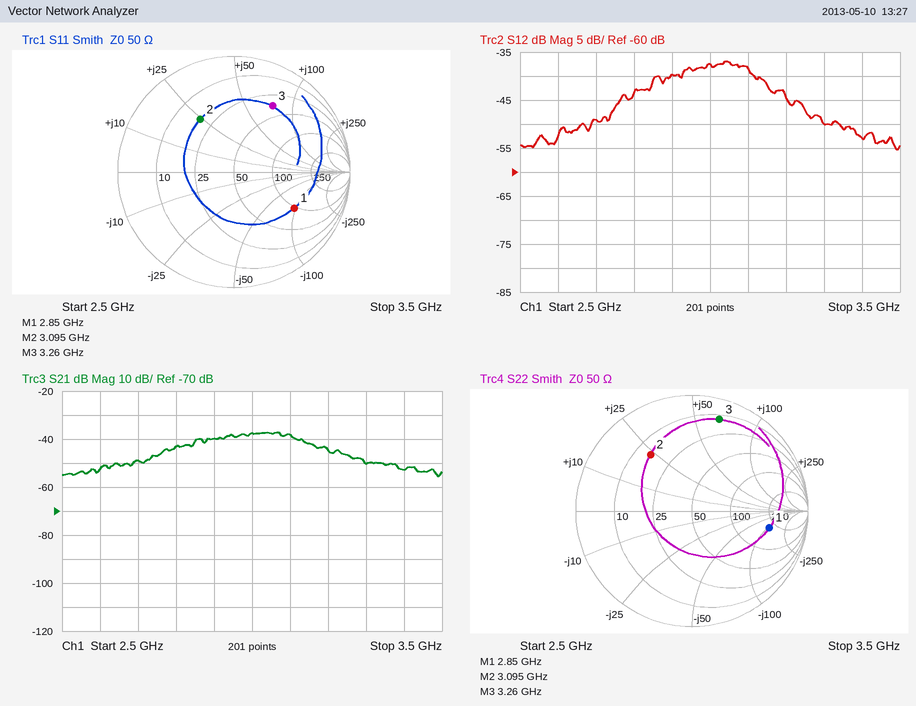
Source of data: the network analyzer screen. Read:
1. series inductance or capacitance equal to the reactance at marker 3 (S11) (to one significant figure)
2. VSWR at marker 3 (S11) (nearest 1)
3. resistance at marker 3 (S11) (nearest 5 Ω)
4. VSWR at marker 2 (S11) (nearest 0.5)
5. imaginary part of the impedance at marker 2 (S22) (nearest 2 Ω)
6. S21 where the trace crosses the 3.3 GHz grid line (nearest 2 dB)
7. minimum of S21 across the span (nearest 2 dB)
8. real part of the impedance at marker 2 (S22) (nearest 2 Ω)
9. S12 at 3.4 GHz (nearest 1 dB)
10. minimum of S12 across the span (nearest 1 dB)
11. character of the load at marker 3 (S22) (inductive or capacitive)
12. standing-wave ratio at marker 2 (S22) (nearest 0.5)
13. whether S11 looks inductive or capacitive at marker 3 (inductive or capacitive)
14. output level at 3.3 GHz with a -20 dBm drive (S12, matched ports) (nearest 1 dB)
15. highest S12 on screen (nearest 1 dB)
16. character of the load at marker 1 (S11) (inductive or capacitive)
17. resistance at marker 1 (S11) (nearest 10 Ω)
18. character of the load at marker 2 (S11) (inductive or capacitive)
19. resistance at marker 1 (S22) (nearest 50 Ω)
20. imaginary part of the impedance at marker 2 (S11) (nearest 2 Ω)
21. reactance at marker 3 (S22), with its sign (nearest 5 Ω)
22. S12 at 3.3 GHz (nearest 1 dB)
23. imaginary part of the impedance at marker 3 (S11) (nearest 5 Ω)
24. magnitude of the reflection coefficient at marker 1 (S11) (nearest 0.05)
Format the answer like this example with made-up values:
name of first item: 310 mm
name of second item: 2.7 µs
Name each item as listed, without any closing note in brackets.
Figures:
series inductance or capacitance equal to the reactance at marker 3 (S11): 4 nH
VSWR at marker 3 (S11): 5
resistance at marker 3 (S11): 35 Ω
VSWR at marker 2 (S11): 3.5
imaginary part of the impedance at marker 2 (S22): +24 Ω
S21 where the trace crosses the 3.3 GHz grid line: -50 dB
minimum of S21 across the span: -56 dB
real part of the impedance at marker 2 (S22): 16 Ω
S12 at 3.4 GHz: -53 dB
minimum of S12 across the span: -55 dB
character of the load at marker 3 (S22): inductive
standing-wave ratio at marker 2 (S22): 4.0
whether S11 looks inductive or capacitive at marker 3: inductive
output level at 3.3 GHz with a -20 dBm drive (S12, matched ports): -70 dBm
highest S12 on screen: -37 dB
character of the load at marker 1 (S11): capacitive
resistance at marker 1 (S11): 100 Ω
character of the load at marker 2 (S11): inductive
resistance at marker 1 (S22): 200 Ω
imaginary part of the impedance at marker 2 (S11): +24 Ω
reactance at marker 3 (S22), with its sign: +65 Ω
S12 at 3.3 GHz: -50 dB
imaginary part of the impedance at marker 3 (S11): +75 Ω
magnitude of the reflection coefficient at marker 1 (S11): 0.60
